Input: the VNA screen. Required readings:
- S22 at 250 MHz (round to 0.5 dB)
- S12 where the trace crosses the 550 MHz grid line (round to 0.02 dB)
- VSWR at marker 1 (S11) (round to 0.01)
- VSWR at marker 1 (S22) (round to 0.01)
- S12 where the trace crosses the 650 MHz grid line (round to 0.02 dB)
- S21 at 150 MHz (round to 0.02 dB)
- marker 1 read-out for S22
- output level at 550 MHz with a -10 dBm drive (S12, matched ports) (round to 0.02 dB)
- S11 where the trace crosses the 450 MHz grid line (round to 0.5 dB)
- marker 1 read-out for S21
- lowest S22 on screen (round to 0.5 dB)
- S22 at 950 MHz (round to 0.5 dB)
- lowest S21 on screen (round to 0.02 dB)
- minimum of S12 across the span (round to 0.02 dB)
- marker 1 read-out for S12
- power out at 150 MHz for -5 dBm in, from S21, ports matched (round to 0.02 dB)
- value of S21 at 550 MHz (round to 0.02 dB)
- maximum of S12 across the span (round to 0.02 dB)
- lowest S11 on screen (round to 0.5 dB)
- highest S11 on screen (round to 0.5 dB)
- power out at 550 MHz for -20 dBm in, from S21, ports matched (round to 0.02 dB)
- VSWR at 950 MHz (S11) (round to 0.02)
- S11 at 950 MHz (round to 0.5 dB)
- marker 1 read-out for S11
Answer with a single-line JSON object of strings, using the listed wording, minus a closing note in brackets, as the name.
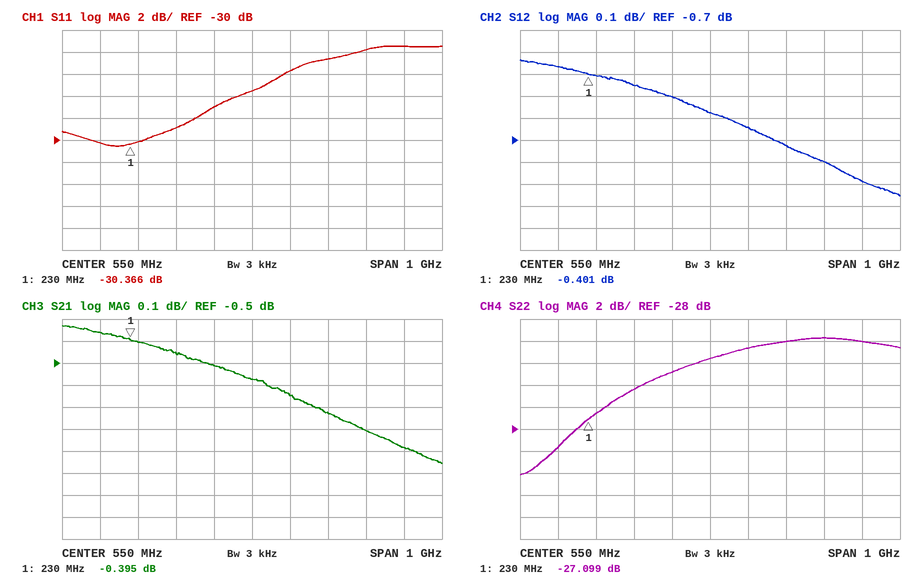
{"S22 at 250 MHz": "-26.5 dB", "S12 where the trace crosses the 550 MHz grid line": "-0.58 dB", "VSWR at marker 1 (S11)": "1.06", "VSWR at marker 1 (S22)": "1.09", "S12 where the trace crosses the 650 MHz grid line": "-0.64 dB", "S21 at 150 MHz": "-0.36 dB", "marker 1 read-out for S22": "-27.099 dB", "output level at 550 MHz with a -10 dBm drive (S12, matched ports)": "-10.58 dBm", "S11 where the trace crosses the 450 MHz grid line": "-27.0 dB", "marker 1 read-out for S21": "-0.395 dB", "lowest S22 on screen": "-32.0 dB", "S22 at 950 MHz": "-20.0 dB", "lowest S21 on screen": "-0.96 dB", "minimum of S12 across the span": "-0.96 dB", "marker 1 read-out for S12": "-0.401 dB", "power out at 150 MHz for -5 dBm in, from S21, ports matched": "-5.36 dBm", "value of S21 at 550 MHz": "-0.58 dB", "maximum of S12 across the span": "-0.34 dB", "lowest S11 on screen": "-30.5 dB", "highest S11 on screen": "-21.5 dB", "power out at 550 MHz for -20 dBm in, from S21, ports matched": "-20.58 dBm", "VSWR at 950 MHz (S11)": "1.18", "S11 at 950 MHz": "-21.5 dB", "marker 1 read-out for S11": "-30.366 dB"}
